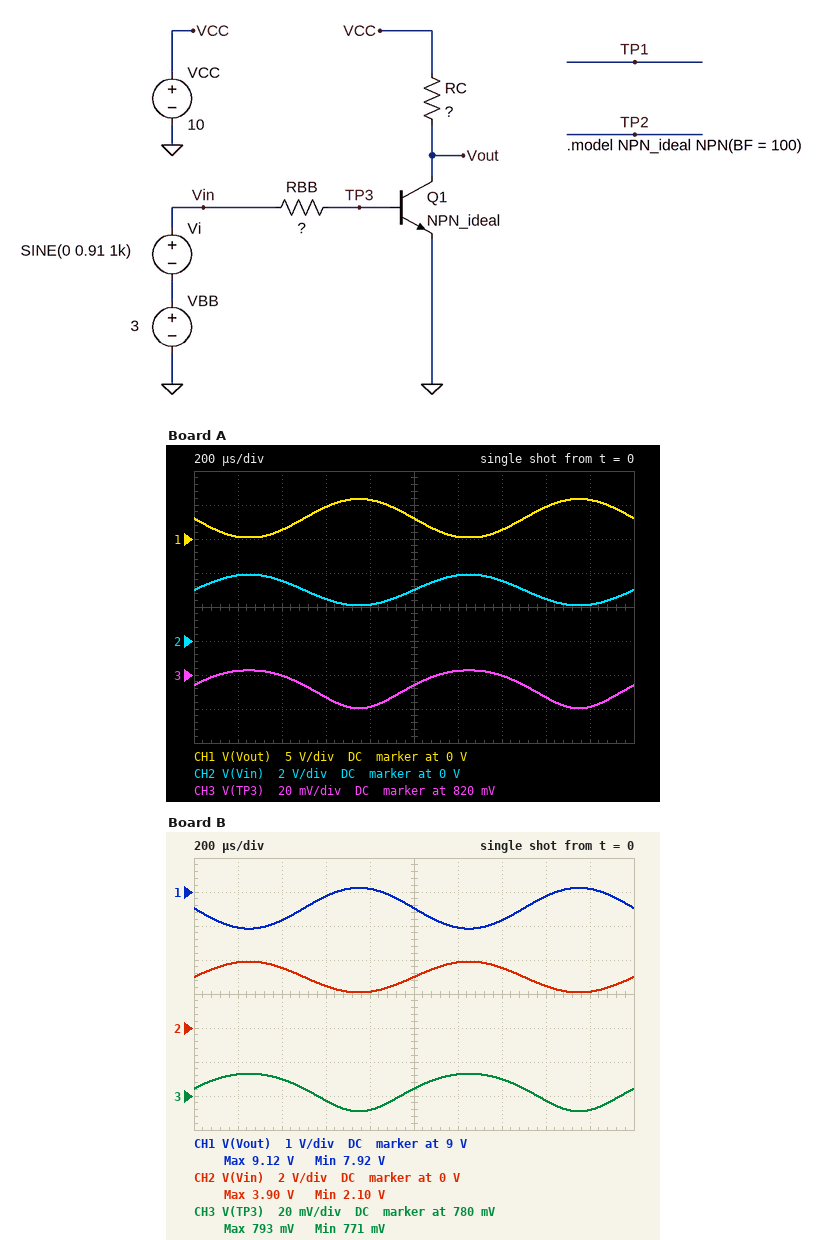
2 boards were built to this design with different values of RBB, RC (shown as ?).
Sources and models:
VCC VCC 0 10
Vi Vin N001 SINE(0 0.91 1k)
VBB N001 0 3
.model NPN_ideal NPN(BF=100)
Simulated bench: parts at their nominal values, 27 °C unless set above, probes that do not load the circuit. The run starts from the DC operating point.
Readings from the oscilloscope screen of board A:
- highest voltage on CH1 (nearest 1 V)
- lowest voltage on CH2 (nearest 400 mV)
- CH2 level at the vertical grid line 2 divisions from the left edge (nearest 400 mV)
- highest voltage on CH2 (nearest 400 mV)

6 V
2.0 V
3.6 V
4.0 V
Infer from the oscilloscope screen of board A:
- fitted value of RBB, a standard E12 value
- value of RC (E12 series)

47 kΩ
1.5 kΩ
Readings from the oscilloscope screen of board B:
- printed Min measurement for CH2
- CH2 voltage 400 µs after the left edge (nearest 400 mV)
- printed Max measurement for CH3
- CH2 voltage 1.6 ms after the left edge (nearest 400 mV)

2.10 V
3.6 V
793 mV
2.4 V
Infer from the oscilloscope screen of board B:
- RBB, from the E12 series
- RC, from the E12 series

150 kΩ
1 kΩ
